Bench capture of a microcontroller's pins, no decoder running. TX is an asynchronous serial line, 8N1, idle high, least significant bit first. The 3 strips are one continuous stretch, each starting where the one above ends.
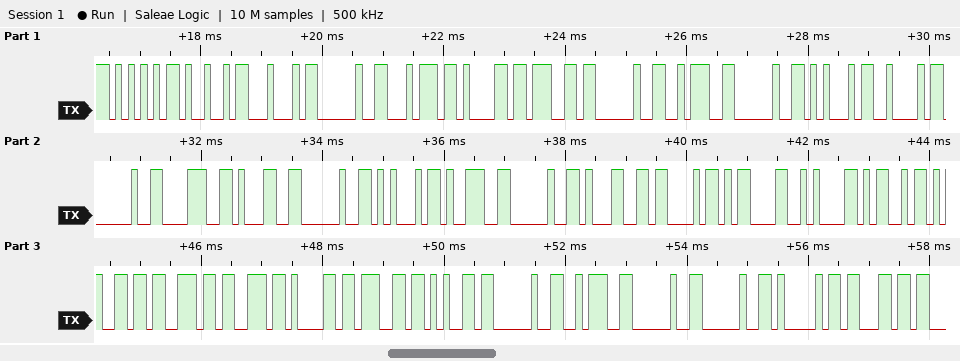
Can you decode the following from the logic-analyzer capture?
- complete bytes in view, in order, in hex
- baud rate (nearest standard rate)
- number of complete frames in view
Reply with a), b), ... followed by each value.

a) 55 49 44 20 74 61 67 20 3A 20 45 42 20 38 31 20 45 39 20 31 43 0D 0A 4D 65 73 73 61 67 65 20 3A 20 20 41 63
b) 9600 baud
c) 36
